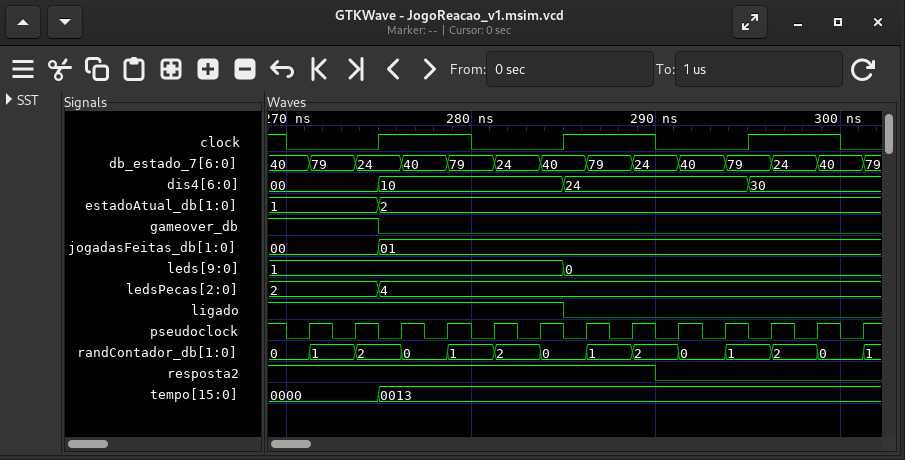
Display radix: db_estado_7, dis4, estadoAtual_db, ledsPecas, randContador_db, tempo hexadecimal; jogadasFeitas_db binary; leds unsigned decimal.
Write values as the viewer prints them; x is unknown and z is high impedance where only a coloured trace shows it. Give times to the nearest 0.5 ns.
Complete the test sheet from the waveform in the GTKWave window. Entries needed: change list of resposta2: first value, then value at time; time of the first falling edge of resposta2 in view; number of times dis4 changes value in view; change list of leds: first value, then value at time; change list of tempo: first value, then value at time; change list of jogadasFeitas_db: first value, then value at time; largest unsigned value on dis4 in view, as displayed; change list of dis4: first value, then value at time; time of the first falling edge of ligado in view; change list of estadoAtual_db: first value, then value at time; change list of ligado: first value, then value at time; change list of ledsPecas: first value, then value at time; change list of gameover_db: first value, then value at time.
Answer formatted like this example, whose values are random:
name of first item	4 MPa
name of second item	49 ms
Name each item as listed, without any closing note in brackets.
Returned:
change list of resposta2: first value, then value at time	1, 0 at 290 ns
time of the first falling edge of resposta2 in view	290 ns
number of times dis4 changes value in view	3
change list of leds: first value, then value at time	1, 0 at 285 ns
change list of tempo: first value, then value at time	0000, 0013 at 275 ns
change list of jogadasFeitas_db: first value, then value at time	00, 01 at 275 ns
largest unsigned value on dis4 in view, as displayed	30
change list of dis4: first value, then value at time	00, 10 at 275 ns, 24 at 285 ns, 30 at 295 ns
time of the first falling edge of ligado in view	285 ns
change list of estadoAtual_db: first value, then value at time	1, 2 at 275 ns
change list of ligado: first value, then value at time	1, 0 at 285 ns
change list of ledsPecas: first value, then value at time	2, 4 at 275 ns
change list of gameover_db: first value, then value at time	1, 0 at 275 ns
